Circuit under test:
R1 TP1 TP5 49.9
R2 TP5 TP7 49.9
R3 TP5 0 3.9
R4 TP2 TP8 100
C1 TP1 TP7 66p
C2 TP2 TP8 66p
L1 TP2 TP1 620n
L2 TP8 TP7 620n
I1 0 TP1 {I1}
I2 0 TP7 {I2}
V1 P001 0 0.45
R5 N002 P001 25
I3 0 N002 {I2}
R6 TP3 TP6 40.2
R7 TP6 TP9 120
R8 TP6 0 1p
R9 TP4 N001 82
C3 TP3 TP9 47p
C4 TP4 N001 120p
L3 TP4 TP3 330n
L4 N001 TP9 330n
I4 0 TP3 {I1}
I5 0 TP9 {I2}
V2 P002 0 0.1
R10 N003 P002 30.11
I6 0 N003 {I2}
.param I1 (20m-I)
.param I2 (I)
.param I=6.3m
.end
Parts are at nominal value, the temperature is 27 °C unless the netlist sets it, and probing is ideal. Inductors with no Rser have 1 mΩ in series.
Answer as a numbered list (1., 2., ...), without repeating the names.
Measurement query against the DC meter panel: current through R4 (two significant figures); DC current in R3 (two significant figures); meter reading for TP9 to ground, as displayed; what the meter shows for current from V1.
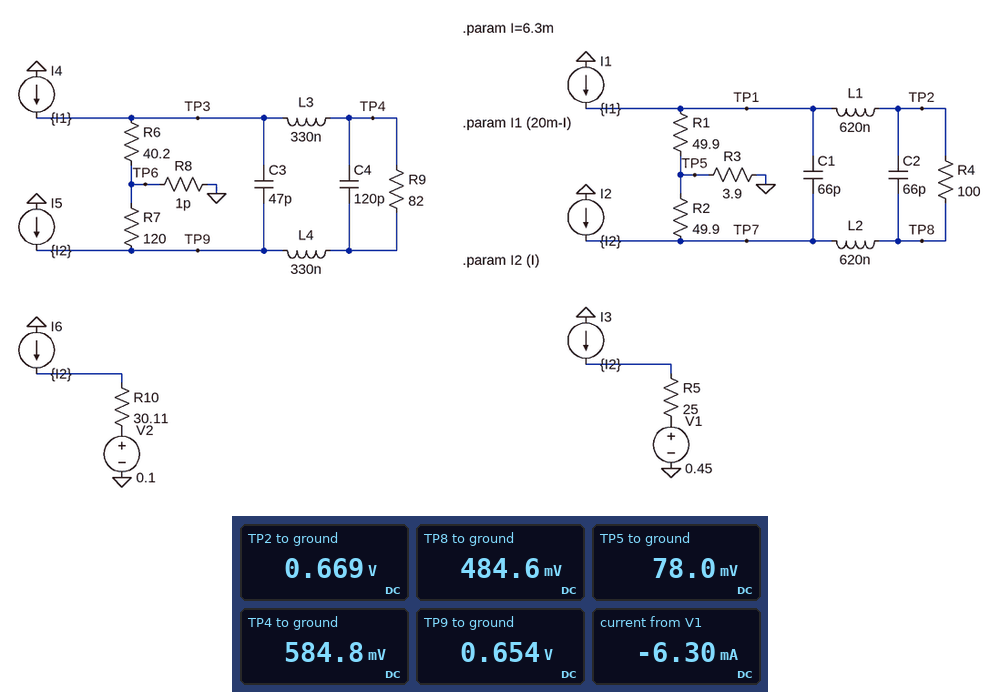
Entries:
1. 1.8 mA
2. 20 mA
3. 0.654 V
4. -6.30 mA
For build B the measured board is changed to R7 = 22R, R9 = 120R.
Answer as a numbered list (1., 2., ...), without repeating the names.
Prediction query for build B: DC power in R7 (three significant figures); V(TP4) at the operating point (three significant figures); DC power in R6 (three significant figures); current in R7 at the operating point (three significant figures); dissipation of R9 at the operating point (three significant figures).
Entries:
1. 1.61 mW
2. 460 mV
3. 5.26 mW
4. 8.56 mA
5. 614 µW
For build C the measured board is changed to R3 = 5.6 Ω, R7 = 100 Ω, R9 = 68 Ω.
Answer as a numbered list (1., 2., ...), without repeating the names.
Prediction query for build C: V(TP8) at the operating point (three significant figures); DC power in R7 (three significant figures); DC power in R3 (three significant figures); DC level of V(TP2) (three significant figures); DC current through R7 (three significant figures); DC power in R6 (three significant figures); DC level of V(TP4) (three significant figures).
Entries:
1. 519 mV
2. 3.50 mW
3. 2.24 mW
4. 703 mV
5. 5.92 mA
6. 7.97 mW
7. 566 mV
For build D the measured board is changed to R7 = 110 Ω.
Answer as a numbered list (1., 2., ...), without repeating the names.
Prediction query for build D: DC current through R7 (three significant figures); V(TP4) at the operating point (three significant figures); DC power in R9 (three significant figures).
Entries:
1. 5.69 mA
2. 575 mV
3. 30.8 µW
